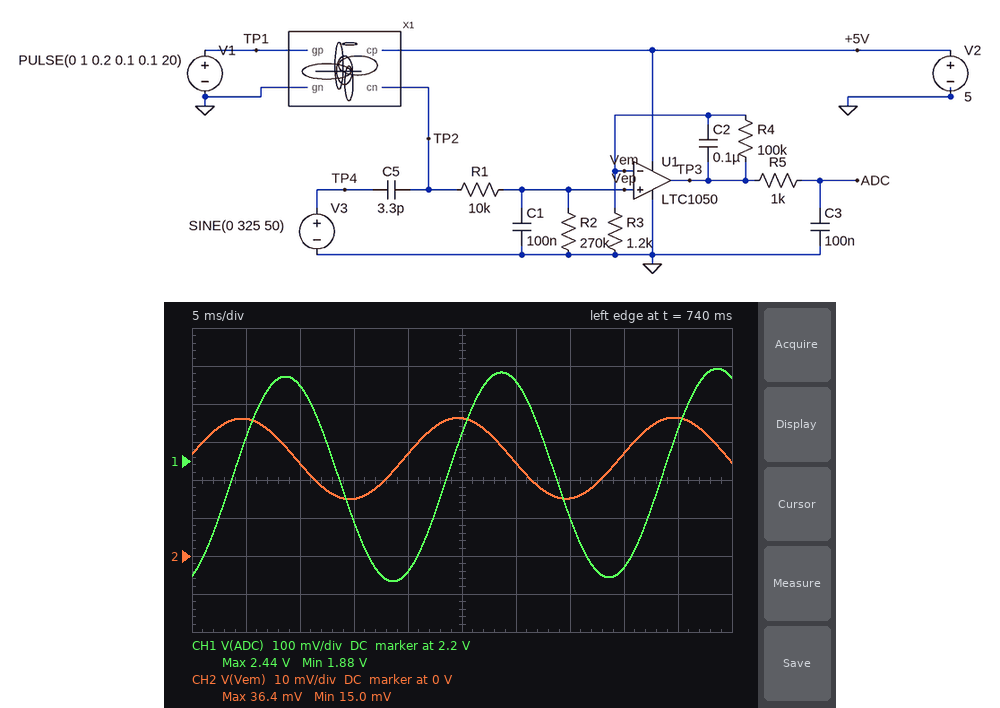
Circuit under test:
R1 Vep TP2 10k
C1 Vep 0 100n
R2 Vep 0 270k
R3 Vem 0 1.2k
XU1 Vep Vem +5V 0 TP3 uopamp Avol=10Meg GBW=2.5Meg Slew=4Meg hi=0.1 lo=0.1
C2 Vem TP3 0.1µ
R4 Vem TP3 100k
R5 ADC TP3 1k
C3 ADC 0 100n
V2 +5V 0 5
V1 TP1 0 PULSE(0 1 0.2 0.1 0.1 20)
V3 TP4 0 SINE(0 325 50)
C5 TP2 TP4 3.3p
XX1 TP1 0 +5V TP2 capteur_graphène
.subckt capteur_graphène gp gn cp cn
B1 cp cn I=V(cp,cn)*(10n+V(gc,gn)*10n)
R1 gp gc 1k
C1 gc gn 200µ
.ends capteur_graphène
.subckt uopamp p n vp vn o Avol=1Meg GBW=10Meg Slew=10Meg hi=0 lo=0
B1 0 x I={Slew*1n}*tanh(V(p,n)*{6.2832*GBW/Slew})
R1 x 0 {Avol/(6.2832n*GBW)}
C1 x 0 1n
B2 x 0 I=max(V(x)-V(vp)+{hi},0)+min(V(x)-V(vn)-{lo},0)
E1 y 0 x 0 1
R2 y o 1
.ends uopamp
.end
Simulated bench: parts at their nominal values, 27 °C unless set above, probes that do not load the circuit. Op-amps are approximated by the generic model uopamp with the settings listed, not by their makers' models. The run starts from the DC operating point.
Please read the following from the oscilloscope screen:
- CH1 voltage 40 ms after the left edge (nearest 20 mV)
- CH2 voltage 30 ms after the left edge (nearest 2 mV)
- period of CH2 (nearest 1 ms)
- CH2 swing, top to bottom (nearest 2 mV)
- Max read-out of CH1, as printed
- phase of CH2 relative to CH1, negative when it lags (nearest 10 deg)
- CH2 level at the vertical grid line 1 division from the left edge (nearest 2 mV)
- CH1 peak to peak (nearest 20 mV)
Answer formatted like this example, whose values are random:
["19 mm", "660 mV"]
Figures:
["1.92 V", "24 mV", "20 ms", "22 mV", "2.44 V", "70 deg", "36 mV", "560 mV"]
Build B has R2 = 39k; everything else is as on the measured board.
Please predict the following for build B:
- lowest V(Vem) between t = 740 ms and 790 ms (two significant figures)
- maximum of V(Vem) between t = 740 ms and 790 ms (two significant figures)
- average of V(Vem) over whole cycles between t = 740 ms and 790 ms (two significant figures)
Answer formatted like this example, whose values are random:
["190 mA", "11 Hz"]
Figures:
["-4.6 mV", "12 mV", "3.7 mV"]
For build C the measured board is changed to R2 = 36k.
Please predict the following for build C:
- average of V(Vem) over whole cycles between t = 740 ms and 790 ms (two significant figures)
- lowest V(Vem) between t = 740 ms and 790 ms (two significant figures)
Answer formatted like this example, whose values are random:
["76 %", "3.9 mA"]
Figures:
["3.5 mV", "-4.6 mV"]
